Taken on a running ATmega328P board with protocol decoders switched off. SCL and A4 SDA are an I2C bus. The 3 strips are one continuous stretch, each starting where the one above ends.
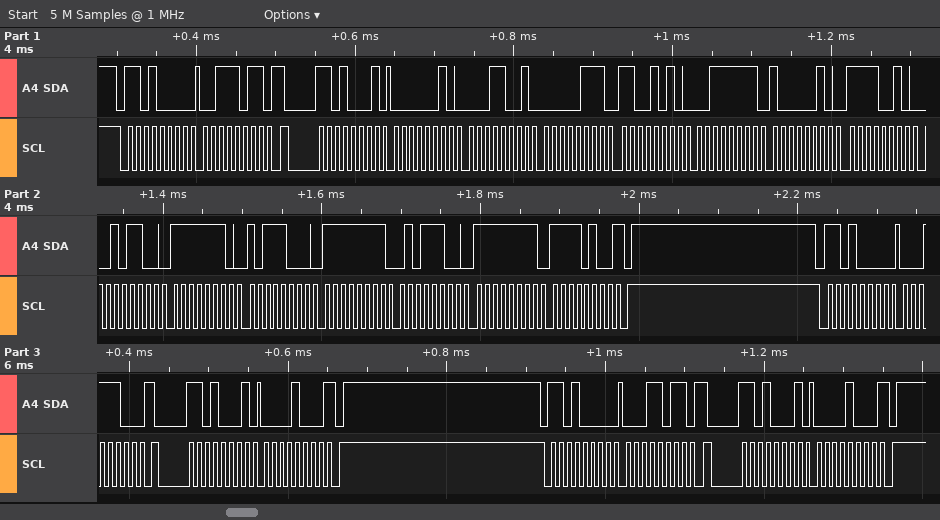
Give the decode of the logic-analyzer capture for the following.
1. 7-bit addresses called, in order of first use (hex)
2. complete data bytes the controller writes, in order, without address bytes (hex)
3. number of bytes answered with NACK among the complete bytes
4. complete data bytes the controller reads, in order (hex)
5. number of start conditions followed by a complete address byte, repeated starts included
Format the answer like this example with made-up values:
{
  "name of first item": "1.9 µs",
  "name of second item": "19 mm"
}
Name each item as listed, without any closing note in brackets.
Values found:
{
  "7-bit addresses called, in order of first use": "0x68",
  "complete data bytes the controller writes, in order, without address bytes": "3B 1C 1B",
  "number of bytes answered with NACK among the complete bytes": "3",
  "complete data bytes the controller reads, in order": "02 19 07 CA 3F 82 F2 2C FE B8 FF 5C FF F4 08 08",
  "number of start conditions followed by a complete address byte, repeated starts included": "6"
}
